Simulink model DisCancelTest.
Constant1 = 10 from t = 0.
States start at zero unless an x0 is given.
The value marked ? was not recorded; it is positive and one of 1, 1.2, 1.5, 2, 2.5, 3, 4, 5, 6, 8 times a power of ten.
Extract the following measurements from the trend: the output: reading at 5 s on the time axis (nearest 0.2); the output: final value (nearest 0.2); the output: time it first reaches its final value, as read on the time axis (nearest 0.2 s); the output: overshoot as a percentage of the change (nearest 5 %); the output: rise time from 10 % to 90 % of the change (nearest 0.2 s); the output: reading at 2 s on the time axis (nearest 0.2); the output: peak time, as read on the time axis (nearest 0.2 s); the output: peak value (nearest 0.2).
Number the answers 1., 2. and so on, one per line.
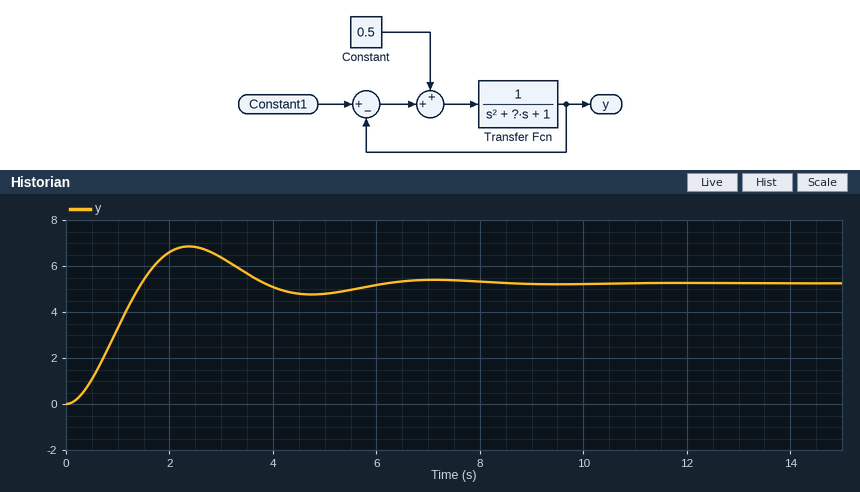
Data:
1. 4.8
2. 5.2
3. 1.4 s
4. 30 %
5. 1.0 s
6. 6.6
7. 2.4 s
8. 6.8
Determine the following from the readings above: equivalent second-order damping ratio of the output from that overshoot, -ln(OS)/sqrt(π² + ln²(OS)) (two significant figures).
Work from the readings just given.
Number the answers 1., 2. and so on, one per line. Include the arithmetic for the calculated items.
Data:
1. ln(0.3) = -1.204; 1.204 / sqrt(9.870 + 1.450) = 0.36
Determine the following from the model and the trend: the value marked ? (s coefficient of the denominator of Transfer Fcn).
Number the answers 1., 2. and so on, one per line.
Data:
1. 1
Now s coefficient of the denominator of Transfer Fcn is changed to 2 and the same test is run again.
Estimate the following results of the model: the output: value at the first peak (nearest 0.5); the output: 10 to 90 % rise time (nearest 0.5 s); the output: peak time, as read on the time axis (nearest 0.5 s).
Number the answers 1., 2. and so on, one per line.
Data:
1. 5.5
2. 1.5 s
3. 3.0 s
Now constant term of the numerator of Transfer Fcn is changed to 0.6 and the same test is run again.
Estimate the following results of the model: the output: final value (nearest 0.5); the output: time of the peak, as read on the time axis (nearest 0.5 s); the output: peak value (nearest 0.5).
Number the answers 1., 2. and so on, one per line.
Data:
1. 4.0
2. 2.5 s
3. 5.0
